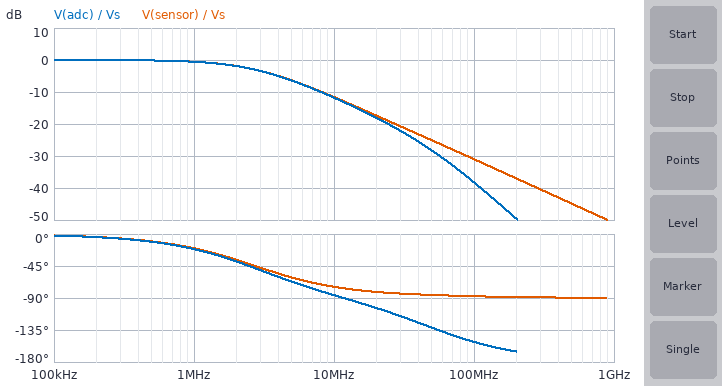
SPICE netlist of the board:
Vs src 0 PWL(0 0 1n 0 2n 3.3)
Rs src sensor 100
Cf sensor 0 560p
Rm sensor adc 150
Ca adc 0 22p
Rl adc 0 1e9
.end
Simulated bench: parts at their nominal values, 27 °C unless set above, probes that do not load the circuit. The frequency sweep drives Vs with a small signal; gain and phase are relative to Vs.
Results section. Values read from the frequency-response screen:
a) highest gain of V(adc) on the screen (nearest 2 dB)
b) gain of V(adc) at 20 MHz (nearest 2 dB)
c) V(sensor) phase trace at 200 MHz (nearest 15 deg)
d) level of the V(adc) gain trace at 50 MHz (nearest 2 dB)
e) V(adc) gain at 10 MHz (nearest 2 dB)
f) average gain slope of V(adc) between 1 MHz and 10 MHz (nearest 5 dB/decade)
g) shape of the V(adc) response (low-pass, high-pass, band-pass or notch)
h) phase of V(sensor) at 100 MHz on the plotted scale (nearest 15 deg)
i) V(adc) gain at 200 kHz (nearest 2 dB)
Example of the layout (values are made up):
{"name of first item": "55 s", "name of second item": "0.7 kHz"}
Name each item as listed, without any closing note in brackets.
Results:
{"highest gain of V(adc) on the screen": "0 dB", "gain of V(adc) at 20 MHz": "-18 dB", "V(sensor) phase trace at 200 MHz": "-90 deg", "level of the V(adc) gain trace at 50 MHz": "-28 dB", "V(adc) gain at 10 MHz": "-12 dB", "average gain slope of V(adc) between 1 MHz and 10 MHz": "-10 dB/decade", "shape of the V(adc) response": "low-pass", "phase of V(sensor) at 100 MHz on the plotted scale": "-90 deg", "V(adc) gain at 200 kHz": "0 dB"}
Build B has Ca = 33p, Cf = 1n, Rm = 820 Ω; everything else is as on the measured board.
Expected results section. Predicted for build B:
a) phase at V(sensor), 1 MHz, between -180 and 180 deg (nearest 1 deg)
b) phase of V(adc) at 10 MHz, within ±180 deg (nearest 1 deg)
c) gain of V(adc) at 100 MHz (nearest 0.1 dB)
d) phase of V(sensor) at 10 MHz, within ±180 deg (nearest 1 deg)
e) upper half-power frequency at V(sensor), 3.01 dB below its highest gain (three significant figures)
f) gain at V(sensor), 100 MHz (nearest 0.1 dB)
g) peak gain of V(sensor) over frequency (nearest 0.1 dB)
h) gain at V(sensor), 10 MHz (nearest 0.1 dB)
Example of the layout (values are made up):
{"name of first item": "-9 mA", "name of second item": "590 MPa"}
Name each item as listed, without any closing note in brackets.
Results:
{"phase at V(sensor), 1 MHz, between -180 and 180 deg": "-33 deg", "phase of V(adc) at 10 MHz, within ±180 deg": "-140 deg", "gain of V(adc) at 100 MHz": "-60.6 dB", "phase of V(sensor) at 10 MHz, within ±180 deg": "-80 deg", "upper half-power frequency at V(sensor), 3.01 dB below its highest gain": "1.53 MHz", "gain at V(sensor), 100 MHz": "-36.0 dB", "peak gain of V(sensor) over frequency": "0 dB", "gain at V(sensor), 10 MHz": "-16.2 dB"}
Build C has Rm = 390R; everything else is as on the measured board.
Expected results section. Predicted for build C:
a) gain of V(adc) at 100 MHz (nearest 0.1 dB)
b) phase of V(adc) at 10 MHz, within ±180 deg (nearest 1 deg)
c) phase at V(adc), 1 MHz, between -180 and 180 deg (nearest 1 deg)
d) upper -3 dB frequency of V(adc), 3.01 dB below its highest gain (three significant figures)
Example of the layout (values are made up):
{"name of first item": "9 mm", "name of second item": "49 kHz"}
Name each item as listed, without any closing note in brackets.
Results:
{"gain of V(adc) at 100 MHz": "-45.7 dB", "phase of V(adc) at 10 MHz, within ±180 deg": "-102 deg", "phase at V(adc), 1 MHz, between -180 and 180 deg": "-23 deg", "upper -3 dB frequency of V(adc), 3.01 dB below its highest gain": "2.67 MHz"}
